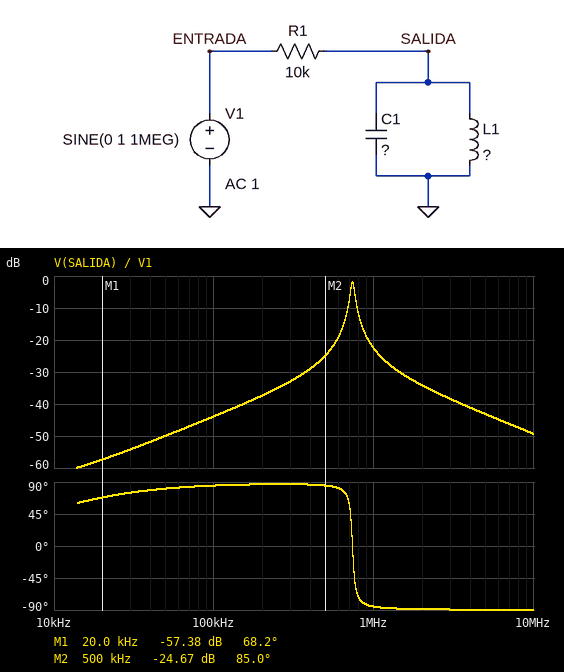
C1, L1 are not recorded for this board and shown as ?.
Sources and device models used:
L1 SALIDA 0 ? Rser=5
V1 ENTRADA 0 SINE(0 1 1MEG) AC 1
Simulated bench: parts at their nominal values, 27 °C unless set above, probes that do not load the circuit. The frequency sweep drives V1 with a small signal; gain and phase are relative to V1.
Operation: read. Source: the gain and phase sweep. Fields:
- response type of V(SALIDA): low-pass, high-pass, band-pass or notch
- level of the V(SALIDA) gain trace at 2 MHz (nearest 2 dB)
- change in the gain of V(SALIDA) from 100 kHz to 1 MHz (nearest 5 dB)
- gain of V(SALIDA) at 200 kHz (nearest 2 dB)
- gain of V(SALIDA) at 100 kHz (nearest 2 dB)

band-pass
-34 dB
20 dB
-38 dB
-44 dB
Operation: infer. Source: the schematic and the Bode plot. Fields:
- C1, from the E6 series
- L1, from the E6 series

470 pF
100 µH
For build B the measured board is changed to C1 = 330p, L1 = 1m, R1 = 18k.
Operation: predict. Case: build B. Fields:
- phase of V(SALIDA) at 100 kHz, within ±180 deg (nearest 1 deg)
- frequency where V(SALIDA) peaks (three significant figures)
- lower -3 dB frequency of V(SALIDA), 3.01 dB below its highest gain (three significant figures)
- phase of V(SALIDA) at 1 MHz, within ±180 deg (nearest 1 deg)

87 deg
277 kHz
264 kHz
-88 deg
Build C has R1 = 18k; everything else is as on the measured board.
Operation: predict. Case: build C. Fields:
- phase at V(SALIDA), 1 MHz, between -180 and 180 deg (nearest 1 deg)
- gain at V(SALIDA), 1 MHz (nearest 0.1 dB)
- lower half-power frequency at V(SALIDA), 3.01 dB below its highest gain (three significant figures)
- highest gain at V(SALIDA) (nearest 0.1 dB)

-87 deg
-27.8 dB
721 kHz
-3.1 dB
